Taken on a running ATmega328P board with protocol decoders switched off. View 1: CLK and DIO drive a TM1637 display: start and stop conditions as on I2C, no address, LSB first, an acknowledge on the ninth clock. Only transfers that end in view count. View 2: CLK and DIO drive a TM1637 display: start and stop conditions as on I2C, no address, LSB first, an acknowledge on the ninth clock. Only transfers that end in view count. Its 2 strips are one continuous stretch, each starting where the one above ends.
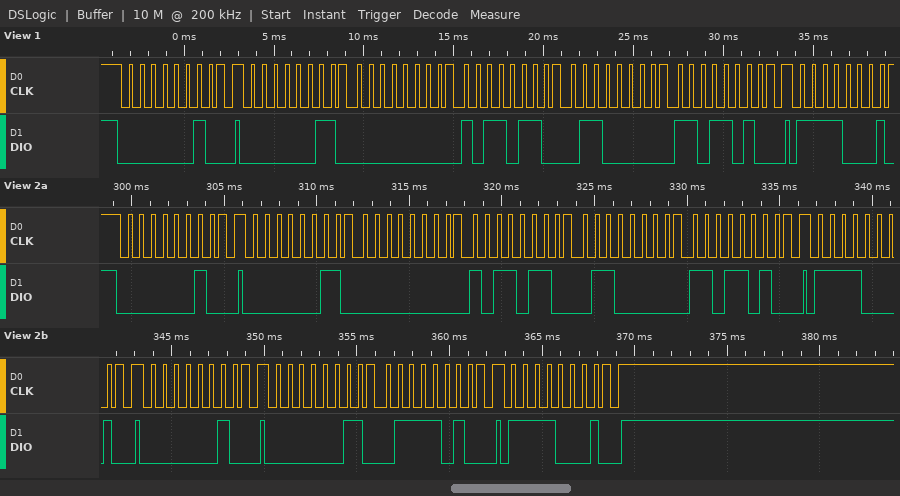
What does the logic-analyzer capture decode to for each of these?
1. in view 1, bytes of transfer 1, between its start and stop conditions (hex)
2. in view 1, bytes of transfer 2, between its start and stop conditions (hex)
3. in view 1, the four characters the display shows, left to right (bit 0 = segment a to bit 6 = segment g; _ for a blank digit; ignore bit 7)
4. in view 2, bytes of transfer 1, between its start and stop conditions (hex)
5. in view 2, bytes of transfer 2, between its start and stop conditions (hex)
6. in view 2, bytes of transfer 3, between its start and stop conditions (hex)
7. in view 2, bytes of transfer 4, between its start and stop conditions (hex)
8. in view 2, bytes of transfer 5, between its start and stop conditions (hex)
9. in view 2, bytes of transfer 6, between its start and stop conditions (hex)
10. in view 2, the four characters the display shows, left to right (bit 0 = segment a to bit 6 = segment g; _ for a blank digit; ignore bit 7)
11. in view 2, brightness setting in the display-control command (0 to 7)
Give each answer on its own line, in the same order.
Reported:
40
C0 00 6D 06 5B
_512
40
C0 00 6D 06 5B
8F
40
C0 5E
8F
d512
7
